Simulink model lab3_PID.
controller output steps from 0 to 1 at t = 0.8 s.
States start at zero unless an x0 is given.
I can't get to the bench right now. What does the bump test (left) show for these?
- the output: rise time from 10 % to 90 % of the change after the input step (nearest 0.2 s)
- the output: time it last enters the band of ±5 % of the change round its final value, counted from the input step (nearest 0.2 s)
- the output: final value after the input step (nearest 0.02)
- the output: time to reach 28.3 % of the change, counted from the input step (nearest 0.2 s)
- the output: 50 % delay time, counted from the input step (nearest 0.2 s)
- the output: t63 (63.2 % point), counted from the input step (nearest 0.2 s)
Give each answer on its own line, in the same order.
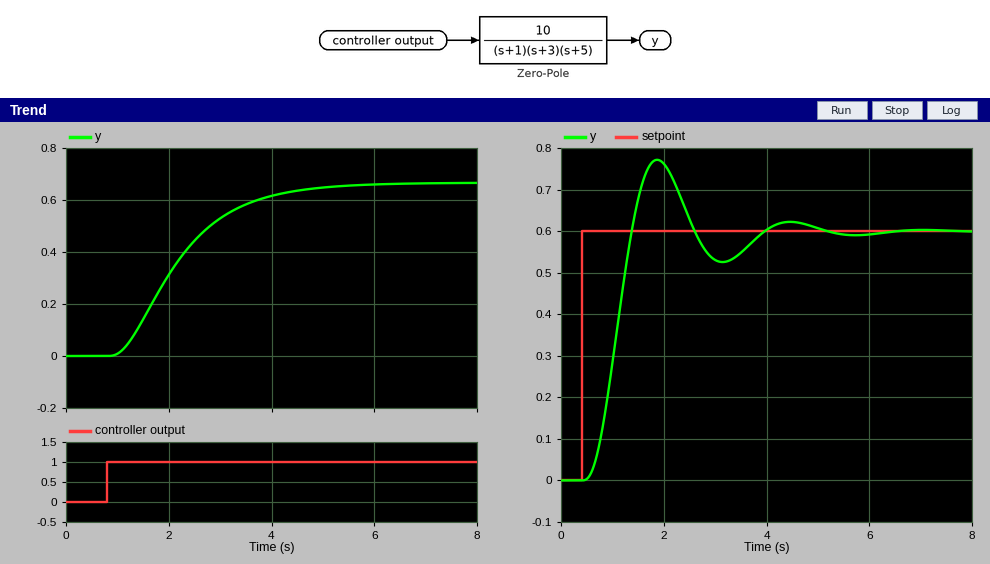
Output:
2.4 s
3.6 s
0.66
0.8 s
1.2 s
1.6 s
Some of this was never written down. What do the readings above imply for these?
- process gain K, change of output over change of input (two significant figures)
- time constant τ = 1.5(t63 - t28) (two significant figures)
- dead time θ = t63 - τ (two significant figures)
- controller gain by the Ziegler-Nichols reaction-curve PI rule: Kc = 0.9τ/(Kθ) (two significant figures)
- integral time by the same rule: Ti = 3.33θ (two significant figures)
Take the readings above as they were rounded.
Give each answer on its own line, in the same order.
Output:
0.66
1.2 s
0.40 s
4.1
1.3 s
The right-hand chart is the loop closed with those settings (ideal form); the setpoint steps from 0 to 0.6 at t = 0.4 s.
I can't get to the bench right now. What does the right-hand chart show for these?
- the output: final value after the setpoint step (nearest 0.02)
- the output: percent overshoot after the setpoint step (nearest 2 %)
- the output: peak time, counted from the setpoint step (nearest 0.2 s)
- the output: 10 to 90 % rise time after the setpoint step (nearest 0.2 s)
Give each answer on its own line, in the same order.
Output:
0.60
28 %
1.4 s
0.6 s
